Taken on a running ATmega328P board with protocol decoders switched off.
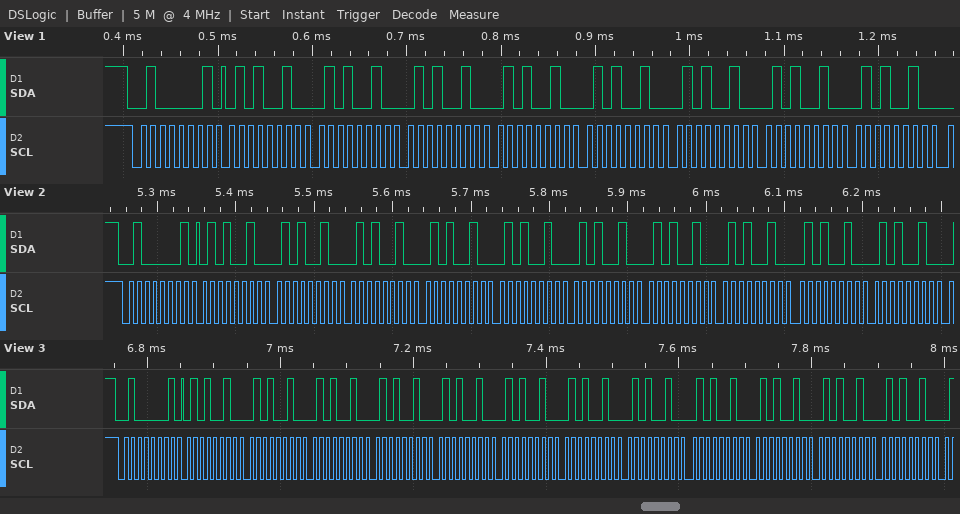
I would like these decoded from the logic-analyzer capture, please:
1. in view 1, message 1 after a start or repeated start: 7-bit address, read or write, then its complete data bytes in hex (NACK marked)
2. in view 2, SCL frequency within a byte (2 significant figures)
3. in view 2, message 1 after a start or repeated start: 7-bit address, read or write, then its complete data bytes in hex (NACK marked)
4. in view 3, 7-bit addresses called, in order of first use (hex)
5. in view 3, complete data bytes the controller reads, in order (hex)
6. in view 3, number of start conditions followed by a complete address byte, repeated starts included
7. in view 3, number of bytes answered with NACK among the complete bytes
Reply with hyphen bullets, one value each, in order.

- 0x20 read: 52 52 52 52 52 52 52 52
- 100 kHz
- 0x20 read: 52 52 52 52 52 52 52 52 52 52
- 0x20
- 52 52 52 52 52 52 52 52 52 52 52 52
- 1
- 0
